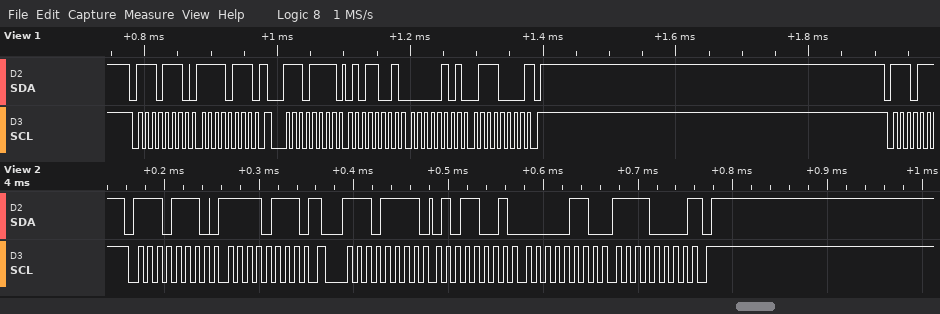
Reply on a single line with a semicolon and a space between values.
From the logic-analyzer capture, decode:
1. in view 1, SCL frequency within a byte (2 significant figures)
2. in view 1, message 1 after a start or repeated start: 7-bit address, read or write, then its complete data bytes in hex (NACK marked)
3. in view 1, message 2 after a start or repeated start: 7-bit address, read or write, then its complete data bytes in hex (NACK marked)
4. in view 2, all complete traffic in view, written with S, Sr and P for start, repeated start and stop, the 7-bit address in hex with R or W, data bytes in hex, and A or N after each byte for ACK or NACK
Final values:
100 kHz; 0x77 write: F7; 0x77 read: 59 05 70 NACK; S 77W A F7 A Sr 77R A 59 A 06 A F0 N P
